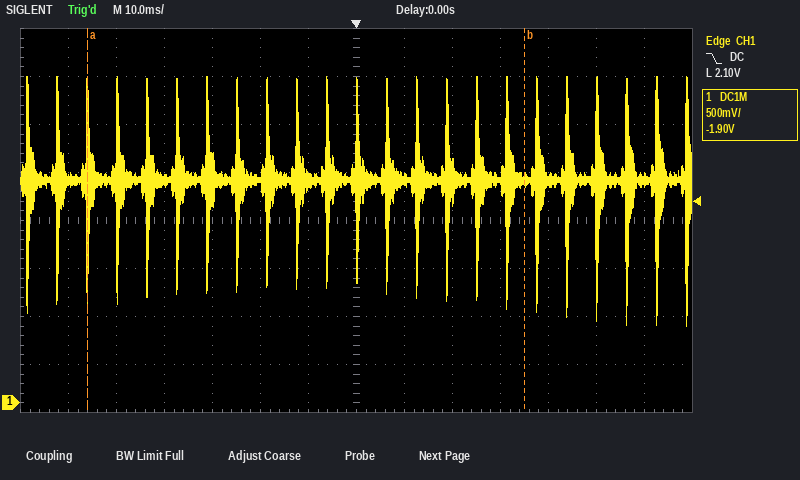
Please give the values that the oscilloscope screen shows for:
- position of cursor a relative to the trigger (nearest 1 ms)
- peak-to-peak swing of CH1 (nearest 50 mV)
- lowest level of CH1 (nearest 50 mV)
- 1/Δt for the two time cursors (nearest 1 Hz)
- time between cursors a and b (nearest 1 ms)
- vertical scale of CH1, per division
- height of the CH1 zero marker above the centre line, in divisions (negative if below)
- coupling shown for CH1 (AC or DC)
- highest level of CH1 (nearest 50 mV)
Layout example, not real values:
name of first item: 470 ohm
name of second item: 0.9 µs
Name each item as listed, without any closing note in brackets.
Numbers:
position of cursor a relative to the trigger: -56 ms
peak-to-peak swing of CH1: 2.60 V
lowest level of CH1: 800 mV
1/Δt for the two time cursors: 11 Hz
time between cursors a and b: 91 ms
vertical scale of CH1, per division: 500 mV
height of the CH1 zero marker above the centre line, in divisions: -3.8 div
coupling shown for CH1: DC
highest level of CH1: 3.40 V
